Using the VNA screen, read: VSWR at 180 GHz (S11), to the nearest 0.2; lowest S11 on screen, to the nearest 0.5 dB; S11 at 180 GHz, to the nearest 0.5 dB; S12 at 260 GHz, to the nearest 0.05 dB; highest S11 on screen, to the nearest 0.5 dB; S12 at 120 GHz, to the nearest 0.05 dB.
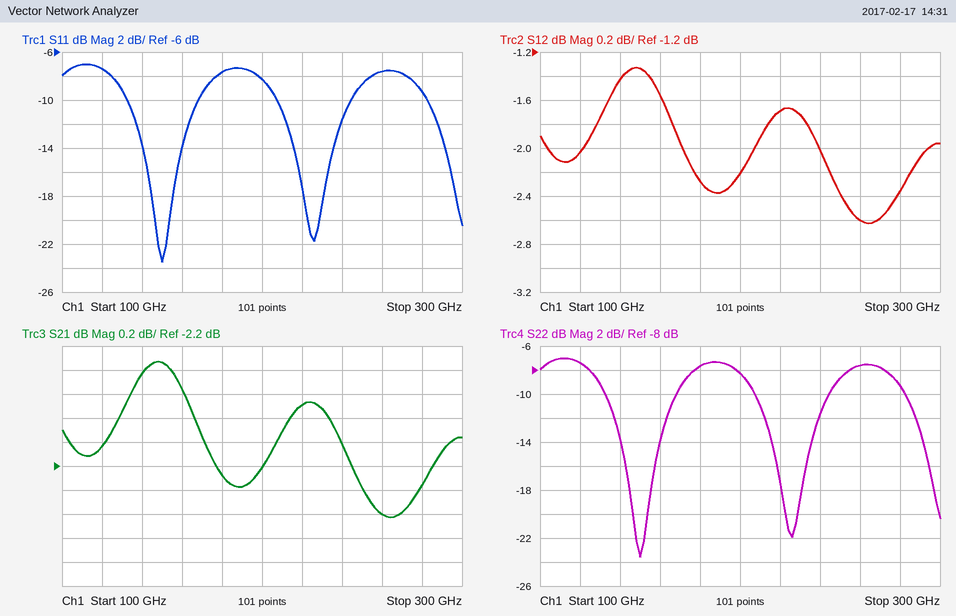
2.4
-23.5 dB
-7.5 dB
-2.60 dB
-7.0 dB
-2.05 dB
